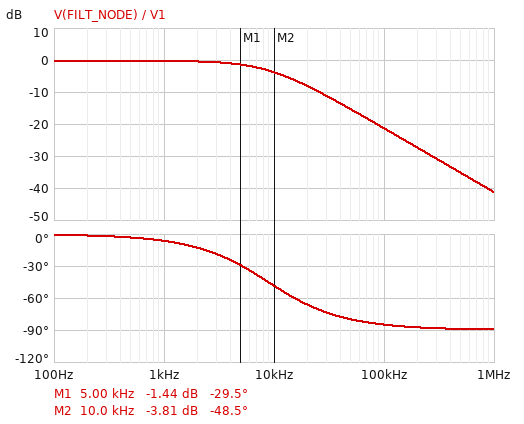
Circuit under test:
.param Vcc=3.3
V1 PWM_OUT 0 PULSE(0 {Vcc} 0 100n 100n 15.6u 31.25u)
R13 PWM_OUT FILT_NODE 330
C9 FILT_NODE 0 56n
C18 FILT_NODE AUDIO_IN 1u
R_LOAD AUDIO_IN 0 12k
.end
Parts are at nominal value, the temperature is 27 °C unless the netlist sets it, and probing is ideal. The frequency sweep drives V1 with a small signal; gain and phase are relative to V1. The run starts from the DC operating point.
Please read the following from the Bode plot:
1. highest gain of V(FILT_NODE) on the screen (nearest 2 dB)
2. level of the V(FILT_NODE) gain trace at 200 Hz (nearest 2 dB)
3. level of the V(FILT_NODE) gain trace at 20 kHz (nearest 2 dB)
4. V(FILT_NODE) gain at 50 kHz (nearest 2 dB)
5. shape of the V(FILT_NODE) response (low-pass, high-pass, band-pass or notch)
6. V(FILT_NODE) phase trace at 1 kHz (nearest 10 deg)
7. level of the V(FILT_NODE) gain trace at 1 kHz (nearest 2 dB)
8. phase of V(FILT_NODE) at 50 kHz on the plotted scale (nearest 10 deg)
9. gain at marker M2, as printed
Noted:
0 dB
0 dB
-8 dB
-16 dB
low-pass
-10 deg
0 dB
-80 deg
-3.81 dB
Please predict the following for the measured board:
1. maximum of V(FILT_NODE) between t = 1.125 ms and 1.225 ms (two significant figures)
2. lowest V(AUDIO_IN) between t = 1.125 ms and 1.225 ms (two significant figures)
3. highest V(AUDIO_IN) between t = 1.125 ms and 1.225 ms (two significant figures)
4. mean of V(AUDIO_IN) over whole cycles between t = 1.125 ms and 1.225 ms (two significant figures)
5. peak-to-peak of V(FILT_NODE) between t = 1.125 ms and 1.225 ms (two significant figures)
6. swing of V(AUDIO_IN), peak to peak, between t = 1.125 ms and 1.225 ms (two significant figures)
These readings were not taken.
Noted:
2.3 V
810 mV
2.1 V
1.5 V
1.3 V
1.3 V
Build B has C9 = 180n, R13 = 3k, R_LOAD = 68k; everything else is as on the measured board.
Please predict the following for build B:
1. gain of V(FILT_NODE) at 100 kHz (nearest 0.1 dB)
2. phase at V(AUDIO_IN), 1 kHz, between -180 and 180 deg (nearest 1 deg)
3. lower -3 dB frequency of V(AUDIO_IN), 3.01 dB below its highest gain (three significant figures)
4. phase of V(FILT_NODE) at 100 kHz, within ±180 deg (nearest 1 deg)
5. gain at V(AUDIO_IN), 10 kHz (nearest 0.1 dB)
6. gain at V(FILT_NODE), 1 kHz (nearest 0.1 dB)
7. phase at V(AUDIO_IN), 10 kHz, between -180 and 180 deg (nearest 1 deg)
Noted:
-50.6 dB
-73 deg
2.21 Hz
-90 deg
-30.6 dB
-11.0 dB
-88 deg
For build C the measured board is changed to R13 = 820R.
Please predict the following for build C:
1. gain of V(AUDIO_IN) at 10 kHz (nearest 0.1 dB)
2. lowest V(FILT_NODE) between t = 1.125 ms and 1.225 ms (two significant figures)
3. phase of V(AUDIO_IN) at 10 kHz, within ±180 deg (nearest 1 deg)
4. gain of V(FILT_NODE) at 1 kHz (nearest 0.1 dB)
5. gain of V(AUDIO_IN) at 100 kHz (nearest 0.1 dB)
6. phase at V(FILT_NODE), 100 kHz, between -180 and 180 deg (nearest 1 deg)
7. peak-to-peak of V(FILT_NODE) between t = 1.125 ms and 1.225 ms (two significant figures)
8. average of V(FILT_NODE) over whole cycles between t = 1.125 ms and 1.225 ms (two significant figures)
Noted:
-9.8 dB
1.3 V
-70 deg
-0.9 dB
-29.2 dB
-88 deg
550 mV
1.6 V
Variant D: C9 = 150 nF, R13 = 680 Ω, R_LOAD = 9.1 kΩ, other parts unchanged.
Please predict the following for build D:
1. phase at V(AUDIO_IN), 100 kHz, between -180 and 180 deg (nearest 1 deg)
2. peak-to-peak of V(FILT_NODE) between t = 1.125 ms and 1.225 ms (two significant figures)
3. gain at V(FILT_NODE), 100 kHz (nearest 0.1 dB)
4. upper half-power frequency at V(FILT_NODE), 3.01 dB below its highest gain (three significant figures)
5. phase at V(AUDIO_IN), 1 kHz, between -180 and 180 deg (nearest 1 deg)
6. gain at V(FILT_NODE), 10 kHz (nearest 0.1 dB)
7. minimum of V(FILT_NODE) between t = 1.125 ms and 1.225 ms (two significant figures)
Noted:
-89 deg
250 mV
-36.1 dB
1.43 kHz
-30 deg
-16.3 dB
1.4 V
